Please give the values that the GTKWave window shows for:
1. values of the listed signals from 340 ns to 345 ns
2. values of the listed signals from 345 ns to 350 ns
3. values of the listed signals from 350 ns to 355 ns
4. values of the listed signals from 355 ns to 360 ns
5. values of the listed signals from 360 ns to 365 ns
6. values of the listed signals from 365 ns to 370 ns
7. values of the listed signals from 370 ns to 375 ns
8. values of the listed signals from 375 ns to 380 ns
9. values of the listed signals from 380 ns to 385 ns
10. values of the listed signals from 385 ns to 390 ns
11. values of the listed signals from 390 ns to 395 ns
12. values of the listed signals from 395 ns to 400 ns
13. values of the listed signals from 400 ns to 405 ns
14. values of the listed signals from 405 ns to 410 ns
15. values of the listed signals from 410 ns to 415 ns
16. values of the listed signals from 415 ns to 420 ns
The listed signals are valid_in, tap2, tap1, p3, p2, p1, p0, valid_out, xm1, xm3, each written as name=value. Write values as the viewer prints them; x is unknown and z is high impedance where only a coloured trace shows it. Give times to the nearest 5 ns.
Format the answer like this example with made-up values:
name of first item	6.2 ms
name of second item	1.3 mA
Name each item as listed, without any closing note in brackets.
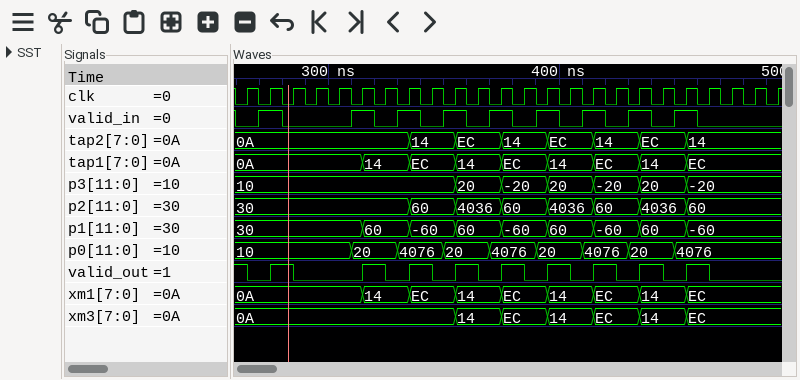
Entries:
values of the listed signals from 340 ns to 345 ns	valid_in=0, tap2=14, tap1=EC, p3=10, p2=60, p1=-60, p0=4076, valid_out=1, xm1=EC, xm3=0A
values of the listed signals from 345 ns to 350 ns	valid_in=0, tap2=14, tap1=EC, p3=10, p2=60, p1=-60, p0=4076, valid_out=0, xm1=EC, xm3=0A
values of the listed signals from 350 ns to 355 ns	valid_in=1, tap2=14, tap1=EC, p3=10, p2=60, p1=-60, p0=20, valid_out=0, xm1=EC, xm3=0A
values of the listed signals from 355 ns to 360 ns	valid_in=1, tap2=EC, tap1=14, p3=20, p2=4036, p1=60, p0=20, valid_out=1, xm1=14, xm3=14
values of the listed signals from 360 ns to 365 ns	valid_in=0, tap2=EC, tap1=14, p3=20, p2=4036, p1=60, p0=20, valid_out=1, xm1=14, xm3=14
values of the listed signals from 365 ns to 370 ns	valid_in=0, tap2=EC, tap1=14, p3=20, p2=4036, p1=60, p0=20, valid_out=0, xm1=14, xm3=14
values of the listed signals from 370 ns to 375 ns	valid_in=1, tap2=EC, tap1=14, p3=20, p2=4036, p1=60, p0=4076, valid_out=0, xm1=14, xm3=14
values of the listed signals from 375 ns to 380 ns	valid_in=1, tap2=14, tap1=EC, p3=-20, p2=60, p1=-60, p0=4076, valid_out=1, xm1=EC, xm3=EC
values of the listed signals from 380 ns to 385 ns	valid_in=0, tap2=14, tap1=EC, p3=-20, p2=60, p1=-60, p0=4076, valid_out=1, xm1=EC, xm3=EC
values of the listed signals from 385 ns to 390 ns	valid_in=0, tap2=14, tap1=EC, p3=-20, p2=60, p1=-60, p0=4076, valid_out=0, xm1=EC, xm3=EC
values of the listed signals from 390 ns to 395 ns	valid_in=1, tap2=14, tap1=EC, p3=-20, p2=60, p1=-60, p0=20, valid_out=0, xm1=EC, xm3=EC
values of the listed signals from 395 ns to 400 ns	valid_in=1, tap2=EC, tap1=14, p3=20, p2=4036, p1=60, p0=20, valid_out=1, xm1=14, xm3=14
values of the listed signals from 400 ns to 405 ns	valid_in=0, tap2=EC, tap1=14, p3=20, p2=4036, p1=60, p0=20, valid_out=1, xm1=14, xm3=14
values of the listed signals from 405 ns to 410 ns	valid_in=0, tap2=EC, tap1=14, p3=20, p2=4036, p1=60, p0=20, valid_out=0, xm1=14, xm3=14
values of the listed signals from 410 ns to 415 ns	valid_in=1, tap2=EC, tap1=14, p3=20, p2=4036, p1=60, p0=4076, valid_out=0, xm1=14, xm3=14
values of the listed signals from 415 ns to 420 ns	valid_in=1, tap2=14, tap1=EC, p3=-20, p2=60, p1=-60, p0=4076, valid_out=1, xm1=EC, xm3=EC
